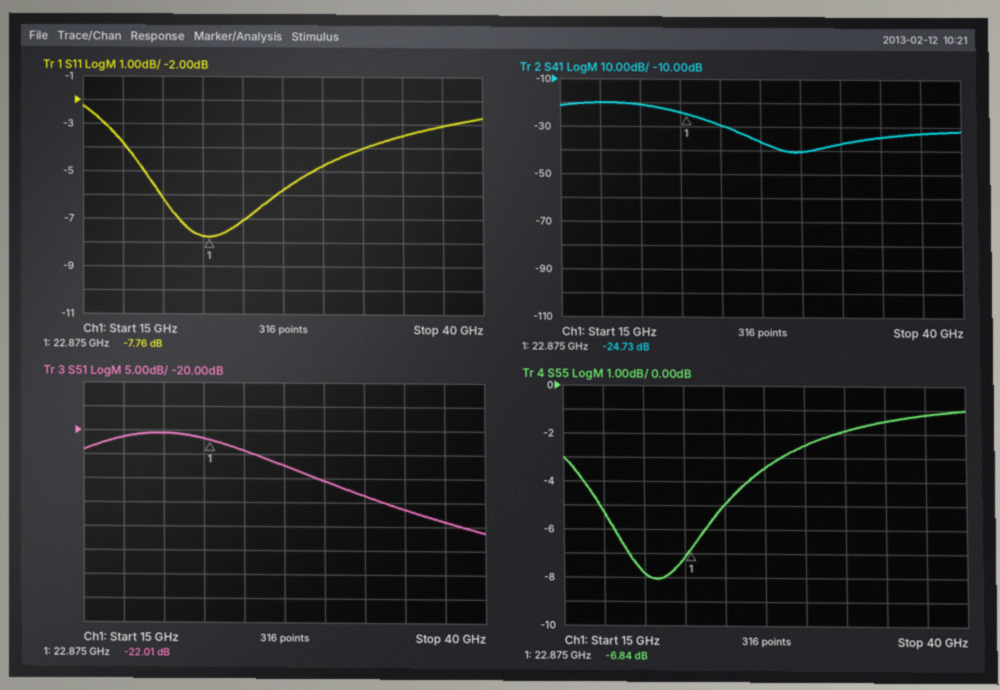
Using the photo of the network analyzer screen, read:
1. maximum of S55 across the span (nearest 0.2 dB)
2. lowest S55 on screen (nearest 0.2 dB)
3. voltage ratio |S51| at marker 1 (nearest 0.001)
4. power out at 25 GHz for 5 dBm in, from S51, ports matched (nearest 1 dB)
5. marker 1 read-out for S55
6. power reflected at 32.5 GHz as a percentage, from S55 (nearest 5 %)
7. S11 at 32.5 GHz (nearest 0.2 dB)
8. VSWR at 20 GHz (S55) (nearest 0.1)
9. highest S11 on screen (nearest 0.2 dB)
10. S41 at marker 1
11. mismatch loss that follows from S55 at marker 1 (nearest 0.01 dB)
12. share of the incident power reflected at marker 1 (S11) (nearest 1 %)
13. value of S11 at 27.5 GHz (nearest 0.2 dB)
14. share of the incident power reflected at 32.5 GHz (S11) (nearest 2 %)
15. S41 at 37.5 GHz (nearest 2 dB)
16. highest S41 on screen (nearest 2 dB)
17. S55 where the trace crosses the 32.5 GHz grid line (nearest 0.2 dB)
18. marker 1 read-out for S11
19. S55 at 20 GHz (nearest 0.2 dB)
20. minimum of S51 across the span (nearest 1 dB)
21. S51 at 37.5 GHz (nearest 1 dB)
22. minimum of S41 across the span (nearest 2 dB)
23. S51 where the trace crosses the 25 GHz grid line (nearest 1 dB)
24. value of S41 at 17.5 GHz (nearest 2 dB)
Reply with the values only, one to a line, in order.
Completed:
-1.0 dB
-8.0 dB
0.079
-19 dBm
-6.84 dB
65 %
-4.0 dB
2.4
-2.2 dB
-24.73 dB
1.01 dB
17 %
-5.8 dB
40 %
-32 dB
-20 dB
-1.8 dB
-7.76 dB
-7.8 dB
-41 dB
-39 dB
-40 dB
-24 dB
-20 dB
